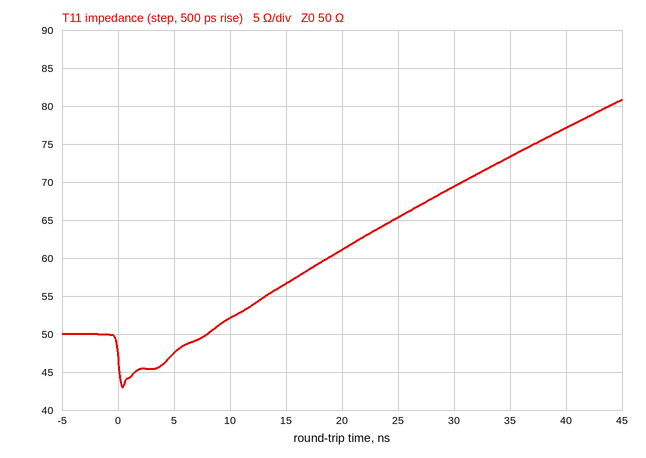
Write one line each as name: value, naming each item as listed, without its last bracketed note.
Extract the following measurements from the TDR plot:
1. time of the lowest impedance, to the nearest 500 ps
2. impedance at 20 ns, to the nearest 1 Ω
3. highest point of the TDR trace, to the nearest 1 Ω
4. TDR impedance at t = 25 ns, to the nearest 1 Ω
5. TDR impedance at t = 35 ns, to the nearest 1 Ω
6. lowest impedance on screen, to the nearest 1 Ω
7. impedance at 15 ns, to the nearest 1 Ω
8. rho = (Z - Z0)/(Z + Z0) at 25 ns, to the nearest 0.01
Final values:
time of the lowest impedance, to the nearest 500 ps: 500 ps
impedance at 20 ns, to the nearest 1 Ω: 61 Ω
highest point of the TDR trace, to the nearest 1 Ω: 81 Ω
TDR impedance at t = 25 ns, to the nearest 1 Ω: 65 Ω
TDR impedance at t = 35 ns, to the nearest 1 Ω: 73 Ω
lowest impedance on screen, to the nearest 1 Ω: 43 Ω
impedance at 15 ns, to the nearest 1 Ω: 57 Ω
rho = (Z - Z0)/(Z + Z0) at 25 ns, to the nearest 0.01: +0.13
